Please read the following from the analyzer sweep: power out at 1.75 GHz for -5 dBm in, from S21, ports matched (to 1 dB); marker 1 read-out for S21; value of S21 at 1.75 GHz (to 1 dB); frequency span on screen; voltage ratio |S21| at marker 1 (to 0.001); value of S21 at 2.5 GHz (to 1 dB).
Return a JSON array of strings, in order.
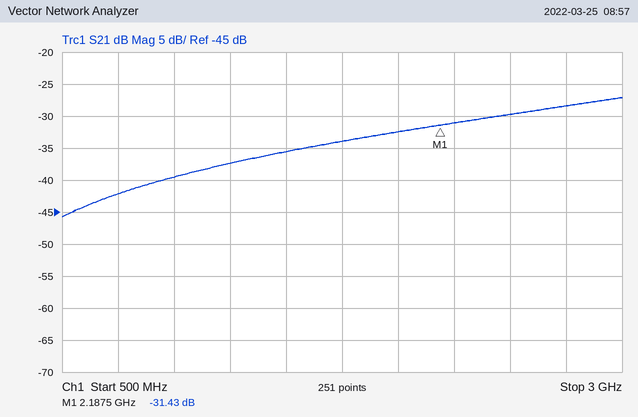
["-39 dBm", "-31.43 dB", "-34 dB", "2.5 GHz", "0.027", "-30 dB"]
